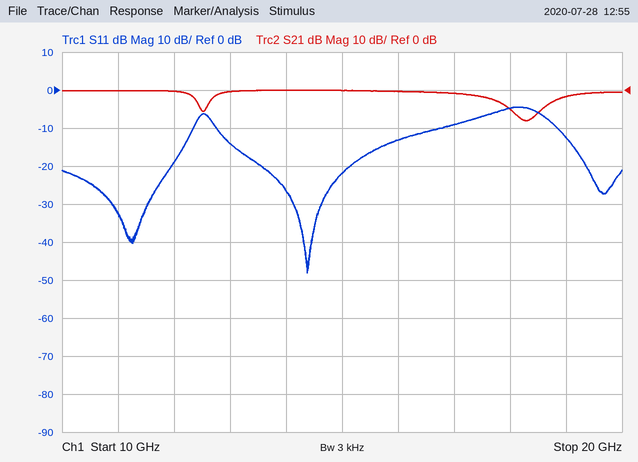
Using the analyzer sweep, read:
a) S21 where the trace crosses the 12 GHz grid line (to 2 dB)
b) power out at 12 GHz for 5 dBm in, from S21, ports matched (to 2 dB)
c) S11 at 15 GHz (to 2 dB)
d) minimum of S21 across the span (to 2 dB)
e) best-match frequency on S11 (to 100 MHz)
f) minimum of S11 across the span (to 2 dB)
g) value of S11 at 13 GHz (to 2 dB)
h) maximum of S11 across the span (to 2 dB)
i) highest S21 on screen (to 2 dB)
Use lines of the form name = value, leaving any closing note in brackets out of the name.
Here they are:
S21 where the trace crosses the 12 GHz grid line = 0 dB
power out at 12 GHz for 5 dBm in, from S21, ports matched = 4 dBm
S11 at 15 GHz = -22 dB
minimum of S21 across the span = -8 dB
best-match frequency on S11 = 14.4 GHz
minimum of S11 across the span = -48 dB
value of S11 at 13 GHz = -14 dB
maximum of S11 across the span = -4 dB
highest S21 on screen = 0 dB
